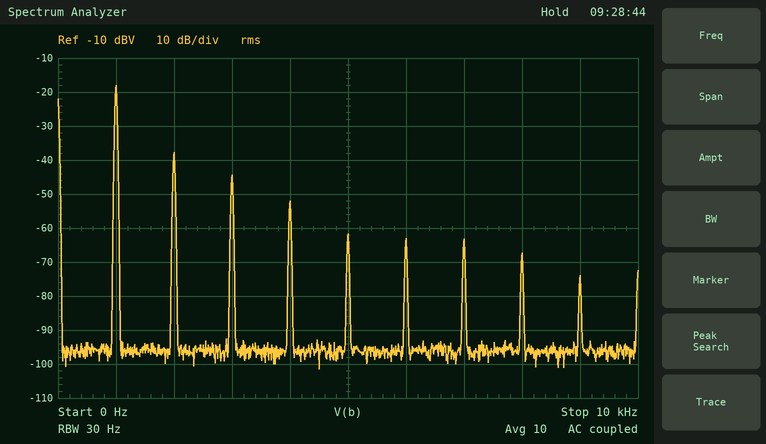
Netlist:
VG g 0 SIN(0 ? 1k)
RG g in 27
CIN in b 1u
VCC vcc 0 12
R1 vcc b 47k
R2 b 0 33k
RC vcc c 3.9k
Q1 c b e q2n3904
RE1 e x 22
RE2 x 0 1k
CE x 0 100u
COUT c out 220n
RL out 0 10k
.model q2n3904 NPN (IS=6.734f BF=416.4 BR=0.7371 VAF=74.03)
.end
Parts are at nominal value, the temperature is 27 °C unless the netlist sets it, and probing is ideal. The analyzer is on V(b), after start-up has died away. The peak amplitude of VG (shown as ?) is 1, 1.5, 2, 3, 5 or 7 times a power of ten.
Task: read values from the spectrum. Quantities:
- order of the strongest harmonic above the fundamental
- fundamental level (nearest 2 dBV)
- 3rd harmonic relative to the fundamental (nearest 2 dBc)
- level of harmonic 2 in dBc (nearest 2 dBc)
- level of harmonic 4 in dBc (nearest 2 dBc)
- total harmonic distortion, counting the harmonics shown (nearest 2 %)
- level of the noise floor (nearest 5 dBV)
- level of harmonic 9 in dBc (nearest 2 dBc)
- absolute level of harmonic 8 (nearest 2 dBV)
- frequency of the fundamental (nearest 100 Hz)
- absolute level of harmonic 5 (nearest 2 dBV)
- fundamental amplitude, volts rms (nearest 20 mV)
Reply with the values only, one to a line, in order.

2
-18 dBV
-26 dBc
-20 dBc
-34 dBc
12 %
-95 dBV
-56 dBc
-68 dBV
1.0 kHz
-62 dBV
120 mV
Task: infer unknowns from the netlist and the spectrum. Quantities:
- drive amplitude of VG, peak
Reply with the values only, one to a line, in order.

200 mV
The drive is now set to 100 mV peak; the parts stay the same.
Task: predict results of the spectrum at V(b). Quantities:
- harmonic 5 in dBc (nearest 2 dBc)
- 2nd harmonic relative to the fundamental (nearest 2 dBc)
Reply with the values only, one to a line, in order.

-38 dBc
-16 dBc
